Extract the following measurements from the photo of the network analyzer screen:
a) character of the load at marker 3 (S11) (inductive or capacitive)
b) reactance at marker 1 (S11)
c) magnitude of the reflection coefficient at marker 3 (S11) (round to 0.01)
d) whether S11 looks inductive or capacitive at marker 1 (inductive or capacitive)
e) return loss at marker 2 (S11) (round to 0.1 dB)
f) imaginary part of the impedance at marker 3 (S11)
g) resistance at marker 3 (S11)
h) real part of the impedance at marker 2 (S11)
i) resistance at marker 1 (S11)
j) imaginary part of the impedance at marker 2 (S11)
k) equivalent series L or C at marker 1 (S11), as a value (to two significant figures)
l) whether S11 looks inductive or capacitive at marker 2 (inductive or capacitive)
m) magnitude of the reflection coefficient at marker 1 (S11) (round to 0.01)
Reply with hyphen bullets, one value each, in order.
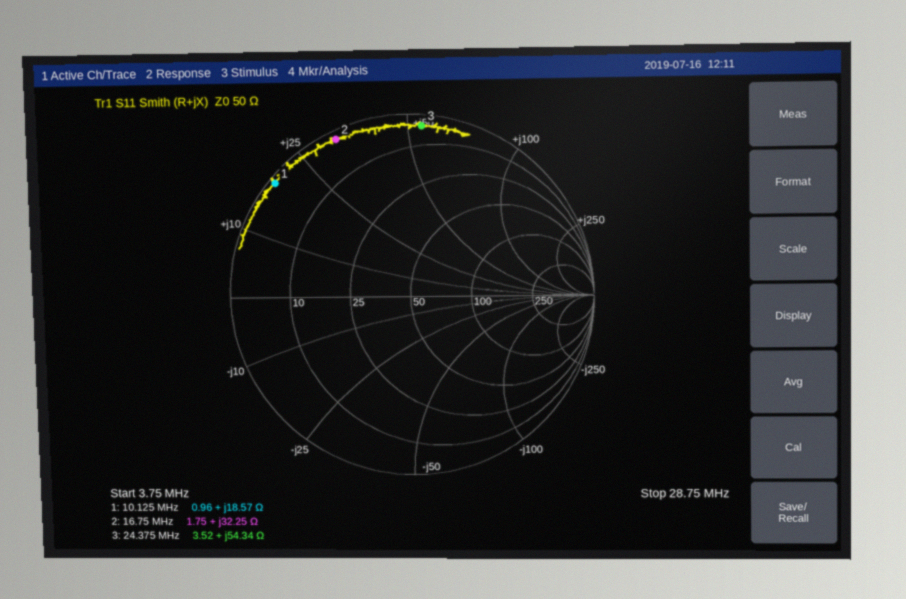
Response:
- inductive
- +18.57 Ω
- 0.94
- inductive
- 0.4 dB
- +54.34 Ω
- 3.52 Ω
- 1.75 Ω
- 0.96 Ω
- +32.25 Ω
- 290 nH
- inductive
- 0.97
